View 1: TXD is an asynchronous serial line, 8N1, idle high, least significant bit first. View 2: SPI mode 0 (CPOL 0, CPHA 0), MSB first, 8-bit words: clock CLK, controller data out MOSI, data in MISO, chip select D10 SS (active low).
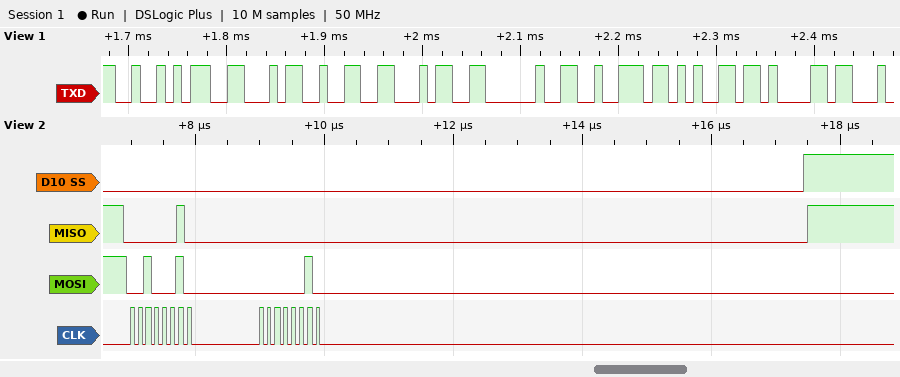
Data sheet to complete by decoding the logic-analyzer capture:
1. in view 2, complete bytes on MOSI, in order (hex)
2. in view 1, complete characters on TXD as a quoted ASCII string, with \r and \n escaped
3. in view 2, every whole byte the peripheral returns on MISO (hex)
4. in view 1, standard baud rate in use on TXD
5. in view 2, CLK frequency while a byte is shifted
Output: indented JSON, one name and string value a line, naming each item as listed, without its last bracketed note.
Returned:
{
  "in view 2, complete bytes on MOSI, in order": "22 02",
  "in view 1, complete characters on TXD as a quoted ASCII string, with \\r and \\n escaped": "\"RF24 rea\"",
  "in view 2, every whole byte the peripheral returns on MISO": "02 00",
  "in view 1, standard baud rate in use on TXD": "115200 baud",
  "in view 2, CLK frequency while a byte is shifted": "8 MHz"
}
